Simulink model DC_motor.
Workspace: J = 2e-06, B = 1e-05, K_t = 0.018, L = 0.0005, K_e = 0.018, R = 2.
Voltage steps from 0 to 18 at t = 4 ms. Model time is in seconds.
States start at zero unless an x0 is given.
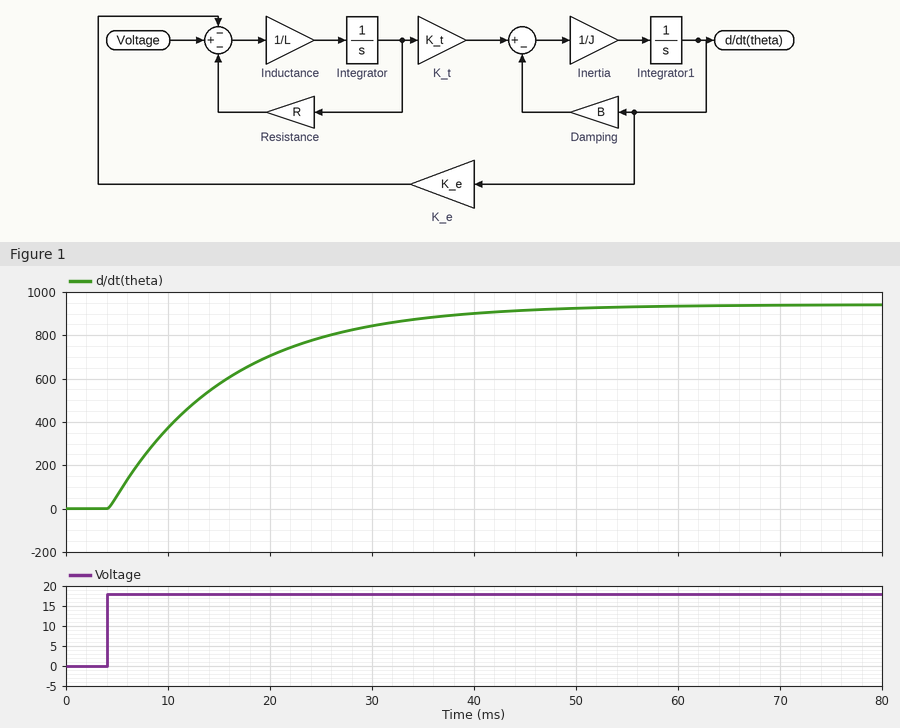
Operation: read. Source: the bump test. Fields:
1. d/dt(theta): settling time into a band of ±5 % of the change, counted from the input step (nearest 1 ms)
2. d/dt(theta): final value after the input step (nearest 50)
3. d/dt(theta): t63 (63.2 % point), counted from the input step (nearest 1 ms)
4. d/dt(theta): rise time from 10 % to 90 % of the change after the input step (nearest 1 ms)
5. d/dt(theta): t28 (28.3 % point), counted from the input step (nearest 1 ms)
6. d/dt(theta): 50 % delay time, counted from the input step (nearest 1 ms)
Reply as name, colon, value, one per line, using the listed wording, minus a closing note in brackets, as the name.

d/dt(theta): settling time into a band of ±5 % of the change, counted from the input step: 34 ms
d/dt(theta): final value after the input step: 950
d/dt(theta): t63 (63.2 % point), counted from the input step: 12 ms
d/dt(theta): rise time from 10 % to 90 % of the change after the input step: 25 ms
d/dt(theta): t28 (28.3 % point), counted from the input step: 4 ms
d/dt(theta): 50 % delay time, counted from the input step: 8 ms
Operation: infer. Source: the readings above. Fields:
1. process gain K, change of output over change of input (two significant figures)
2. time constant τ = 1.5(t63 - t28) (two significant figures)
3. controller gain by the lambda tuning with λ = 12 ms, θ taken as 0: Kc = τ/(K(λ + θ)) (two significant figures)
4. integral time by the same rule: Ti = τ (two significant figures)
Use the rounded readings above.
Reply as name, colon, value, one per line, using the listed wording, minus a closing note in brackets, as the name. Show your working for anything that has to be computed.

process gain K, change of output over change of input: (950 - 0) / 18 = 53
time constant τ = 1.5(t63 - t28): 1.5 × (12 - 4) = 12 ms
controller gain by the lambda tuning with λ = 12 ms, θ taken as 0: Kc = τ/(K(λ + θ)): 12 / (53 × (12 + 0)) = 0.019
integral time by the same rule: Ti = τ: 12 ms
